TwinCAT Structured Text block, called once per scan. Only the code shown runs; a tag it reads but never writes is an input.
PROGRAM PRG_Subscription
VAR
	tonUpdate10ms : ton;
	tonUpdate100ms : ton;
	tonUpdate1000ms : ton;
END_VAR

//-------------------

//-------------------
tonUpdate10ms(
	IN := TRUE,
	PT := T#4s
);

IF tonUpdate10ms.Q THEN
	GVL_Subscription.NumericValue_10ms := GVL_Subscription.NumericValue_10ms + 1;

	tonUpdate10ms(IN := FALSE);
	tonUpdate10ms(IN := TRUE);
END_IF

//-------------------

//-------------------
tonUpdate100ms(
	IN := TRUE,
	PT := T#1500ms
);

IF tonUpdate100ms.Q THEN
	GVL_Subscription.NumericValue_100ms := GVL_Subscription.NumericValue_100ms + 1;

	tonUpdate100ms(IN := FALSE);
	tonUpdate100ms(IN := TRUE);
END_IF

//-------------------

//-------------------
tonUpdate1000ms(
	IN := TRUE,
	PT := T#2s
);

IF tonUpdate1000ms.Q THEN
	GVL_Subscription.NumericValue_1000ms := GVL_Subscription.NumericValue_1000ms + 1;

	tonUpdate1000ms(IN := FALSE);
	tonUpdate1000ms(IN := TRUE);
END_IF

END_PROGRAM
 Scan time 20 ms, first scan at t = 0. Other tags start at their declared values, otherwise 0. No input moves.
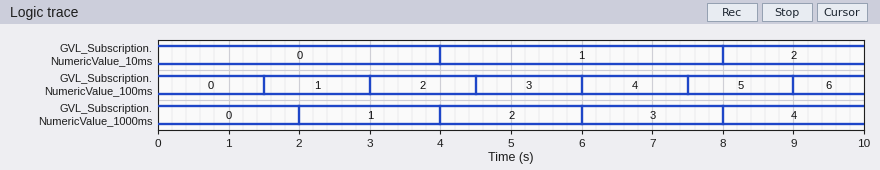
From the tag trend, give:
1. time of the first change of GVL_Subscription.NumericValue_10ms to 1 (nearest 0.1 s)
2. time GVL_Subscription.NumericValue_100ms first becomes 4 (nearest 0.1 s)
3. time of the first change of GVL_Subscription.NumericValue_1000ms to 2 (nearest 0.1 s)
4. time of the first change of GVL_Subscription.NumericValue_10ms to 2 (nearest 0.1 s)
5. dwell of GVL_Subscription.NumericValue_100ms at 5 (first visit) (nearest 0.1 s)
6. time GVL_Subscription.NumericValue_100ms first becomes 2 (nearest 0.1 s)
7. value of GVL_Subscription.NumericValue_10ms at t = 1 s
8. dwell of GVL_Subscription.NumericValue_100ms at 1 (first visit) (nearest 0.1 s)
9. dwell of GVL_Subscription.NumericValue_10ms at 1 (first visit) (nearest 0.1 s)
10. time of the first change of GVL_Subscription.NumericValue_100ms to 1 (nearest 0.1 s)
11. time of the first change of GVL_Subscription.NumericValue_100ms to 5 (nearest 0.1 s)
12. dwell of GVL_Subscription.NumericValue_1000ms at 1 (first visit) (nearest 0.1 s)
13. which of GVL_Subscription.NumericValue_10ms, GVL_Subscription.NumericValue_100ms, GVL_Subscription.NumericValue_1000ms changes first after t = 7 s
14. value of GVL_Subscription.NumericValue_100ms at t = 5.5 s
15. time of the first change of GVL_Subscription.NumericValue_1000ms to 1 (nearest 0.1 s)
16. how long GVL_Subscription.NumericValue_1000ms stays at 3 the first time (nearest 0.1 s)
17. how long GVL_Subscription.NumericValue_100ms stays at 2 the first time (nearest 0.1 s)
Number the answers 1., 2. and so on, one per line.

1. 4.0 s
2. 6.0 s
3. 4.0 s
4. 8.0 s
5. 1.5 s
6. 3.0 s
7. 0
8. 1.5 s
9. 4.0 s
10. 1.5 s
11. 7.5 s
12. 2.0 s
13. GVL_Subscription.NumericValue_100ms
14. 3
15. 2.0 s
16. 2.0 s
17. 1.5 s
